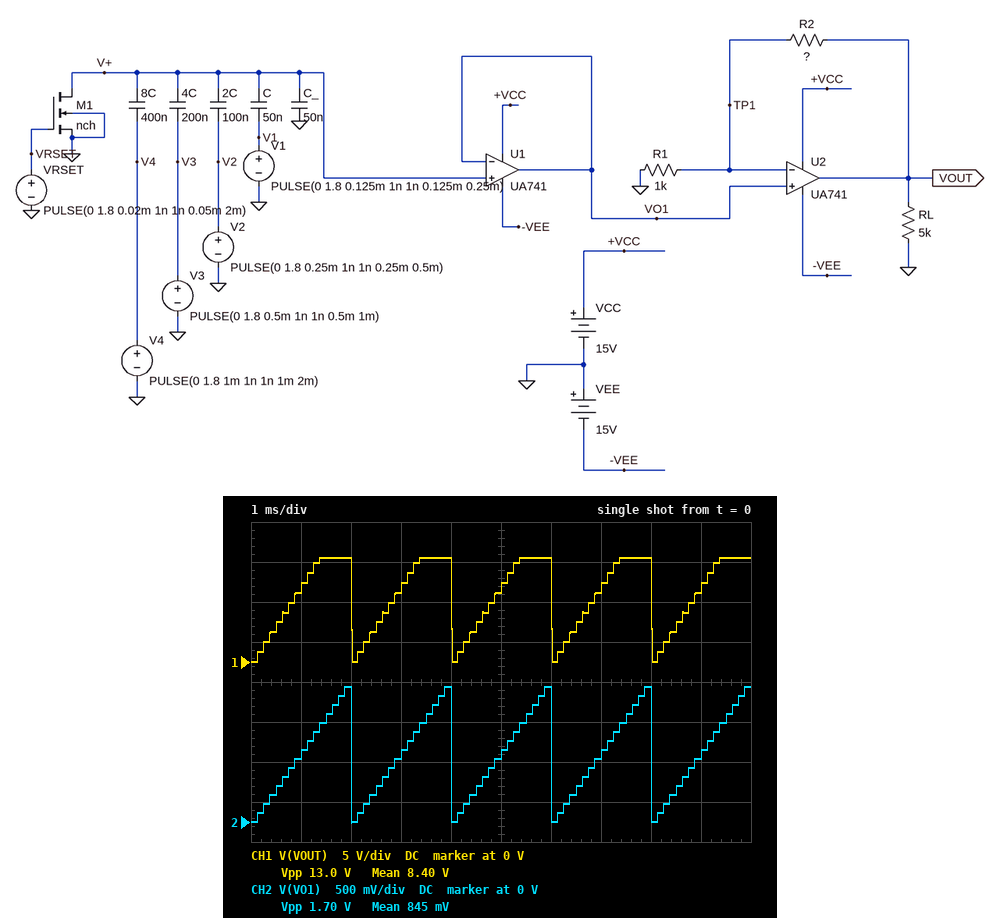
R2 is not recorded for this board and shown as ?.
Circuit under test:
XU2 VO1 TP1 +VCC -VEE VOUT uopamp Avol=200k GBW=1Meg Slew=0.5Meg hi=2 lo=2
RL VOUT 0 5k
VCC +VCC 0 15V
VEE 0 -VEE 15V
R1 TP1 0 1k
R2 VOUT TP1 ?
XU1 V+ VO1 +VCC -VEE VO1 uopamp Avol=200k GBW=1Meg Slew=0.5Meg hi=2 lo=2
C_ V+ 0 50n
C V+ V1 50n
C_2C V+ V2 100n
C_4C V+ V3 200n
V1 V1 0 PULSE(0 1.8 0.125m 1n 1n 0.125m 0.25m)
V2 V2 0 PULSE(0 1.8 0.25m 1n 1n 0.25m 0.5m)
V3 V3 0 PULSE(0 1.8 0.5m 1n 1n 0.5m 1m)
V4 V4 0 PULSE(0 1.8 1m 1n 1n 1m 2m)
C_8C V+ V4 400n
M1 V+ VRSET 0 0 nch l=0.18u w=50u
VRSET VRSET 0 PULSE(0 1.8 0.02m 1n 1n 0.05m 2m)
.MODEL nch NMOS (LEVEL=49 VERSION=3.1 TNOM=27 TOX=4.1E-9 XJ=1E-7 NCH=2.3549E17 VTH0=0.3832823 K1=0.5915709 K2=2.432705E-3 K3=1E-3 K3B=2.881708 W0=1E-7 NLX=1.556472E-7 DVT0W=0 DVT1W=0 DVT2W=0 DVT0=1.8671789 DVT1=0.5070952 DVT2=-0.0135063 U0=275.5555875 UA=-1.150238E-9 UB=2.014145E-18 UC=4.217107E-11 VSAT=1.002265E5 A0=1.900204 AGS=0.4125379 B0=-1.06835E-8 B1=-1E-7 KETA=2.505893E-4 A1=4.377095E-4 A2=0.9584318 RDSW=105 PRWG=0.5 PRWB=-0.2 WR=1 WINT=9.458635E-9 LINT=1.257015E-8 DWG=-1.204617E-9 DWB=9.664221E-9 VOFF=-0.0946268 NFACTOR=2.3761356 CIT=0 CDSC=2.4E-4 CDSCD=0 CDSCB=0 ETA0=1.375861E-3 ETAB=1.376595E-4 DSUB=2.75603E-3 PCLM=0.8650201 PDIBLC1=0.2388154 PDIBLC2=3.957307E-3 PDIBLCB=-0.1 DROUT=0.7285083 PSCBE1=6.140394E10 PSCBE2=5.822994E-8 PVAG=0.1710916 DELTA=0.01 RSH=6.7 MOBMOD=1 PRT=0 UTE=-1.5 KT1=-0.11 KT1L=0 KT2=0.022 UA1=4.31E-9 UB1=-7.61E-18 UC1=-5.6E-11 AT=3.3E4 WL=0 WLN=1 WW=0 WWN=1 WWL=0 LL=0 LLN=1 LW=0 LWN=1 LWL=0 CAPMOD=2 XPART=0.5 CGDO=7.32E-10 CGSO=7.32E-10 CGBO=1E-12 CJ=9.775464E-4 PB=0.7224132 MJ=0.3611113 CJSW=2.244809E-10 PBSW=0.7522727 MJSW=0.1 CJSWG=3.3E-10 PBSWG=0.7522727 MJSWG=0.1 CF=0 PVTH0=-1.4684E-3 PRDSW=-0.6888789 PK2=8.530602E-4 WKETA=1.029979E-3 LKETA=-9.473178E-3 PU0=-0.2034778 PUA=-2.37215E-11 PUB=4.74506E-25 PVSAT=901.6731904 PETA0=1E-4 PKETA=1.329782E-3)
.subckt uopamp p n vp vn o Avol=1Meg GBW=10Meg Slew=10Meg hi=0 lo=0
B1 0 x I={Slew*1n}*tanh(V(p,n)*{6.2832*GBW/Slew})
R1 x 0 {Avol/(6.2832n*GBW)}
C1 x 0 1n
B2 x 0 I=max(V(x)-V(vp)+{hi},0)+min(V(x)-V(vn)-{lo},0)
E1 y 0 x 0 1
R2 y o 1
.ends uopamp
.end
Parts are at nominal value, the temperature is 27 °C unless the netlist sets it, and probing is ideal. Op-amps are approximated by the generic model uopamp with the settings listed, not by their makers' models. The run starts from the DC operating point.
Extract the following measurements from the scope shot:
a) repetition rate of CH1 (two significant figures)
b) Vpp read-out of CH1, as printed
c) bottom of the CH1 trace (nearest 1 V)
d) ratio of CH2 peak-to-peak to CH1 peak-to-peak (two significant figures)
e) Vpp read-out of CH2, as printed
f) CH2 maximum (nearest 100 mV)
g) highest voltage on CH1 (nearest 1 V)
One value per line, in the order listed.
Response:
500 Hz
13.0 V
0 V
0.13
1.70 V
1.7 V
13 V
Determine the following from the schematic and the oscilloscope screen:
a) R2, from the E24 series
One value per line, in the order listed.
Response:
10 kΩ
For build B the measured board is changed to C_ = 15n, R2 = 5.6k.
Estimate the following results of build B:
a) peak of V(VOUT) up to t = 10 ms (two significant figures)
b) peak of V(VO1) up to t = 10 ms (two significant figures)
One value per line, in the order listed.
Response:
12 V
1.8 V
